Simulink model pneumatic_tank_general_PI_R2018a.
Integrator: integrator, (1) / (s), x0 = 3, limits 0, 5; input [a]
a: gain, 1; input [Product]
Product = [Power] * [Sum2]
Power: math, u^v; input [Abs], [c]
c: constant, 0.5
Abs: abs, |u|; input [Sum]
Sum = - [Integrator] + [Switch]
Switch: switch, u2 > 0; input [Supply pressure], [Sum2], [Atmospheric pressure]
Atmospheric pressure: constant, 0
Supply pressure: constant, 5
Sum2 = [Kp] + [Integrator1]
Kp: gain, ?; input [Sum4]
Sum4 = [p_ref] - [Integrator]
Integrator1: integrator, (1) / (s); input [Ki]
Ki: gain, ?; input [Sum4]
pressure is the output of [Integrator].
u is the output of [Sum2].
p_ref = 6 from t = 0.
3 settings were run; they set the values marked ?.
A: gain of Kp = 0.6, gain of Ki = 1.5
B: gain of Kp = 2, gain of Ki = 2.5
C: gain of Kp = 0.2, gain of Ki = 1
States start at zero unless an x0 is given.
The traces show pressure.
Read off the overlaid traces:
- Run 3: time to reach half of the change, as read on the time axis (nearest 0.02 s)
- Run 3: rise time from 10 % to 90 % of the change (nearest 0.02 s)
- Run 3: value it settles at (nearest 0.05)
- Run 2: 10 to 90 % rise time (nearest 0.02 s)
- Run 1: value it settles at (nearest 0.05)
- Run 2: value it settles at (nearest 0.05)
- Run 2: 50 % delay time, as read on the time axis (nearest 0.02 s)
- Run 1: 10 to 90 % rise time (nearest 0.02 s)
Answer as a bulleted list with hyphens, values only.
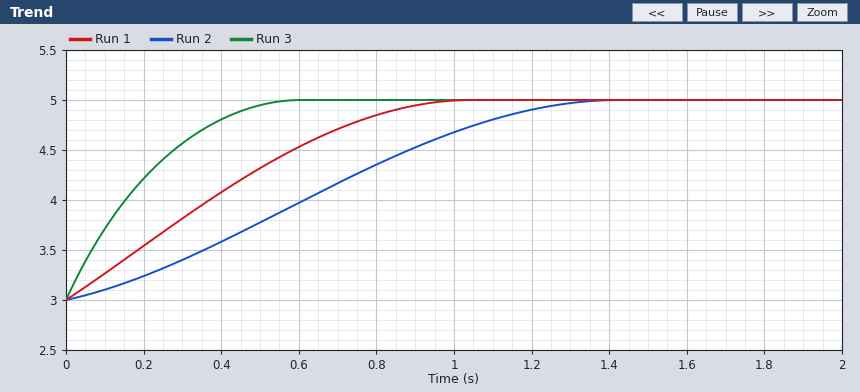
- 0.16 s
- 0.38 s
- 5.00
- 0.92 s
- 5.00
- 5.00
- 0.62 s
- 0.68 s
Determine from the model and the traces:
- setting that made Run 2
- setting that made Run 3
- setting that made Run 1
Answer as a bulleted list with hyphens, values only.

- C
- B
- A
